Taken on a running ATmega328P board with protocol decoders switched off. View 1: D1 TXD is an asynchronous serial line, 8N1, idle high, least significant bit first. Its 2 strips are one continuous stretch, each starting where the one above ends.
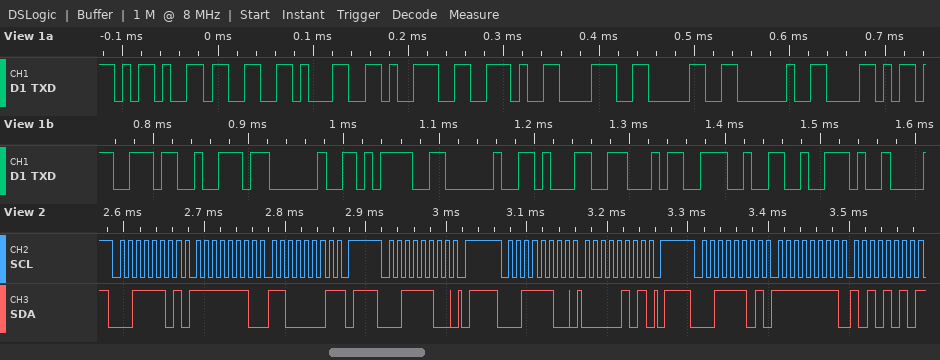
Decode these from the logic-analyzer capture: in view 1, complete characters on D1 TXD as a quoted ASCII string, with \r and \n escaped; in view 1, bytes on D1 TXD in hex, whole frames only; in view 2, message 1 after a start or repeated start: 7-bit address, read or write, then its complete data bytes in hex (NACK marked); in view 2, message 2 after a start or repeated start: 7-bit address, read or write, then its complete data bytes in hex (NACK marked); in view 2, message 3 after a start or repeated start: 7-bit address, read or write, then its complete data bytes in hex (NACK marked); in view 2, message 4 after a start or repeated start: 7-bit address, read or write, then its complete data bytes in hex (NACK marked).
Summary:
"-319.80 Xsr = 142."
2D 33 31 39 2E 38 30 20 58 73 72 20 3D 20 31 34 32 2E
0x1E read: FE C1 NACK
0x1E write
0x1E write: 05
0x1E read: FF AA NACK
